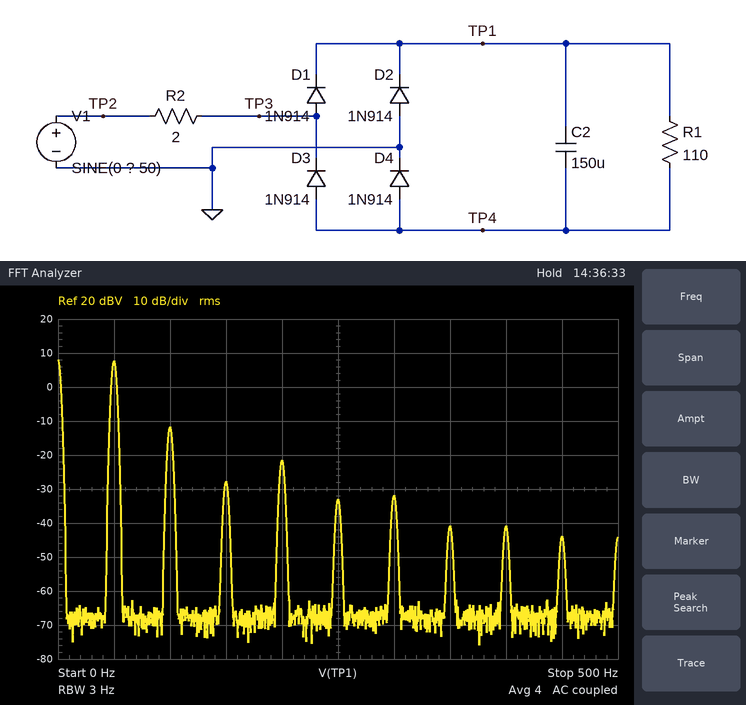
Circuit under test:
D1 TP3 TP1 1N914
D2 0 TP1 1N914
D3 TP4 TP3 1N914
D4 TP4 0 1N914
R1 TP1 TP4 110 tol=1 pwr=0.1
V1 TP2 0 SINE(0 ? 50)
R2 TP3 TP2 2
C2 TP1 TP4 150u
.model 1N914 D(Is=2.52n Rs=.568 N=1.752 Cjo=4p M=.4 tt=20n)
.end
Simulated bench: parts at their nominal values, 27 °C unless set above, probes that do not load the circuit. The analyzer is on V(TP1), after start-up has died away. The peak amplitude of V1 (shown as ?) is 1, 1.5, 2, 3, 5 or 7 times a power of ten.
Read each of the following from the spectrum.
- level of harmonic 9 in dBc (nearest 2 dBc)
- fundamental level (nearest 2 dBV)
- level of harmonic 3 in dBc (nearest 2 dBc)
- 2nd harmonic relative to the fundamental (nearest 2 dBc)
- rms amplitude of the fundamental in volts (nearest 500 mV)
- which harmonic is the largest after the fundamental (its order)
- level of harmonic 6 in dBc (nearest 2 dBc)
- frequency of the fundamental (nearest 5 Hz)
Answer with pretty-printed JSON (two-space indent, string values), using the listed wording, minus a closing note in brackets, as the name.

{
  "level of harmonic 9 in dBc": "-52 dBc",
  "fundamental level": "8 dBV",
  "level of harmonic 3 in dBc": "-36 dBc",
  "2nd harmonic relative to the fundamental": "-20 dBc",
  "rms amplitude of the fundamental in volts": "2.5 V",
  "which harmonic is the largest after the fundamental": "2",
  "level of harmonic 6 in dBc": "-40 dBc",
  "frequency of the fundamental": "50 Hz"
}
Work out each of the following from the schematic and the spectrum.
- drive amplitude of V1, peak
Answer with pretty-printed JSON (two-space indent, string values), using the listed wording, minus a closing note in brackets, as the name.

{
  "drive amplitude of V1, peak": "7 V"
}
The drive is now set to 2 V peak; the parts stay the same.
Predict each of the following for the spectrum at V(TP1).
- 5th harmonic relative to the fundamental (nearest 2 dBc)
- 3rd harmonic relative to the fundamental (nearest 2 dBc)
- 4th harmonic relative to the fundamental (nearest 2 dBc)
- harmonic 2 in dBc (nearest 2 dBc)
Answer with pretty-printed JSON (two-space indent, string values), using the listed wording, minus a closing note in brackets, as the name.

{
  "5th harmonic relative to the fundamental": "-48 dBc",
  "3rd harmonic relative to the fundamental": "-44 dBc",
  "4th harmonic relative to the fundamental": "-38 dBc",
  "harmonic 2 in dBc": "-28 dBc"
}
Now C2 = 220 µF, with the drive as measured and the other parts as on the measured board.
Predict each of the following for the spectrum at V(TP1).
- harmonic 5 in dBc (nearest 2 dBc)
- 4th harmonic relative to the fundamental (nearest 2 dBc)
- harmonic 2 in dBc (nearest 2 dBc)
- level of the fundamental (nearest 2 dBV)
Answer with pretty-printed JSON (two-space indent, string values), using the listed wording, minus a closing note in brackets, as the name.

{
  "harmonic 5 in dBc": "-40 dBc",
  "4th harmonic relative to the fundamental": "-32 dBc",
  "harmonic 2 in dBc": "-22 dBc",
  "level of the fundamental": "8 dBV"
}
